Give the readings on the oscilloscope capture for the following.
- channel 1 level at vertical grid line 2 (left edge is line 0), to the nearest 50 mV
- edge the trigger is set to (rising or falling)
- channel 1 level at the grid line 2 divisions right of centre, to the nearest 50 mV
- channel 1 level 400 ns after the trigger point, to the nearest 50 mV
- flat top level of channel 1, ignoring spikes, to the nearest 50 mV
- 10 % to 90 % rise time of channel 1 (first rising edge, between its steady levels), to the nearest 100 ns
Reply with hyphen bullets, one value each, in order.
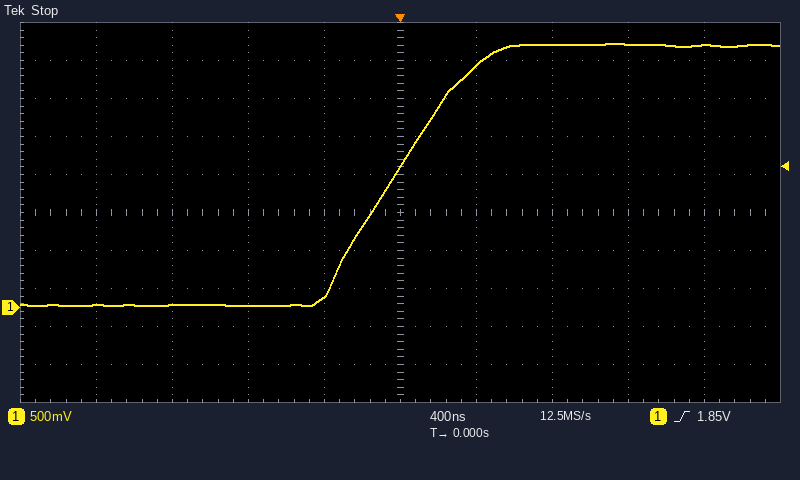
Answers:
- 50 mV
- rising
- 3.45 V
- 3.20 V
- 3.45 V
- 700 ns
